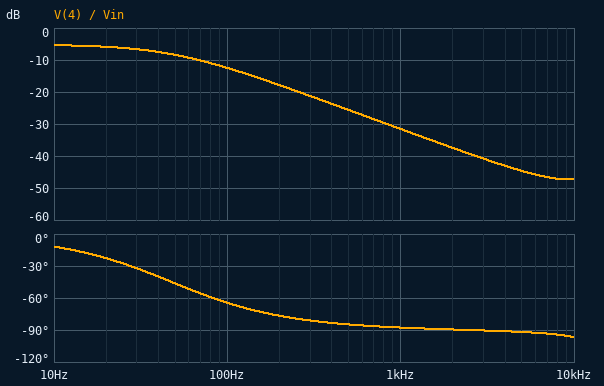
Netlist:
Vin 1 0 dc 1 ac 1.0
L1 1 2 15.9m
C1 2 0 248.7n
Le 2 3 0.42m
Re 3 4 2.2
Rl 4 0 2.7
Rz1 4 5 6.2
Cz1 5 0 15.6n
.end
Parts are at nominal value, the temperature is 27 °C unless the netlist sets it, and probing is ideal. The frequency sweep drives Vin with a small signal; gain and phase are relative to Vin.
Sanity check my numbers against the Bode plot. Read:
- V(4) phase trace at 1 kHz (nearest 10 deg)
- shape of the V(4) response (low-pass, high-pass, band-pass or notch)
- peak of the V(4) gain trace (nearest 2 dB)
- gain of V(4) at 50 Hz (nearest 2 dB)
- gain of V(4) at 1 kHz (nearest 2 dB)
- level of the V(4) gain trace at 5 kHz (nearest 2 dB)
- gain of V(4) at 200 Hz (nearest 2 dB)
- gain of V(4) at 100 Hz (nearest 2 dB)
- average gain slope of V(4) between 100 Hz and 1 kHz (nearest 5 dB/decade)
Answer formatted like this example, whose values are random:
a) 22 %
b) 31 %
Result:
a) -90 deg
b) low-pass
c) -6 dB
d) -8 dB
e) -32 dB
f) -44 dB
g) -18 dB
h) -12 dB
i) -20 dB/decade
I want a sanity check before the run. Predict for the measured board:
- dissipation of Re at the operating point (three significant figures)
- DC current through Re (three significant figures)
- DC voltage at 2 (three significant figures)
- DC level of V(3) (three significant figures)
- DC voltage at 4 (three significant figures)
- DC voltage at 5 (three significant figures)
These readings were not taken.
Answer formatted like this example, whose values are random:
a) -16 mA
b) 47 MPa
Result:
a) 91.6 mW
b) 204 mA
c) 1.00 V
d) 1.00 V
e) 551 mV
f) 551 mV
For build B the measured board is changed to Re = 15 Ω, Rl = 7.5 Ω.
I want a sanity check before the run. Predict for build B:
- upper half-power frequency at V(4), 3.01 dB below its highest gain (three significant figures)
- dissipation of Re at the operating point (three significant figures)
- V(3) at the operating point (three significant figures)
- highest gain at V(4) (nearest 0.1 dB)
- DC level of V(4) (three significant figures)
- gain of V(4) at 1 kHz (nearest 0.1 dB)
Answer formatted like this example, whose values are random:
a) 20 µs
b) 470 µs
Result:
a) 221 Hz
b) 29.6 mW
c) 1.00 V
d) -9.5 dB
e) 333 mV
f) -22.8 dB
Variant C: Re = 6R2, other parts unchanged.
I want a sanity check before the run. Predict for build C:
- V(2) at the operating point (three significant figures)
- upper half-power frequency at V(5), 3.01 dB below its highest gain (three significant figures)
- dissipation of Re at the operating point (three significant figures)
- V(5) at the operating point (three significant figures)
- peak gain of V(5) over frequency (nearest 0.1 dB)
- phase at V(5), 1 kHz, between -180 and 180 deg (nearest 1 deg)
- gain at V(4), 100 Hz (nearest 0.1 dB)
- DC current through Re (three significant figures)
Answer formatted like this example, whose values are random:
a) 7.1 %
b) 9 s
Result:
a) 1.00 V
b) 86.9 Hz
c) 78.3 mW
d) 303 mV
e) -10.4 dB
f) -86 deg
g) -14.0 dB
h) 112 mA
